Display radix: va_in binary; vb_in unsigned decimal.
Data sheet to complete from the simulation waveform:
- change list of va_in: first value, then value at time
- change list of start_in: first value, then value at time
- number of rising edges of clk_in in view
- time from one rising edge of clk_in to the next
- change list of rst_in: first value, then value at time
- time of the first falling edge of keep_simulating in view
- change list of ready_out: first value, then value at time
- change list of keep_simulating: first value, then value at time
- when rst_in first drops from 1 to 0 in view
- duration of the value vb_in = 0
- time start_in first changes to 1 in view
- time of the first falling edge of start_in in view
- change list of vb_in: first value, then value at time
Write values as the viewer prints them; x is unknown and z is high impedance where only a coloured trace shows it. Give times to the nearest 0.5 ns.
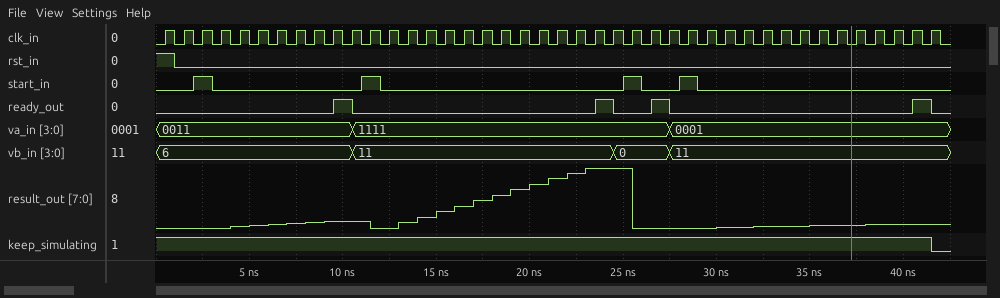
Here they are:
0011, 1111 at 10.5 ns, 0001 at 27.5 ns
0, 1 at 2 ns, 0 at 3 ns, 1 at 11 ns, 0 at 12 ns, 1 at 25 ns, 0 at 26 ns, 1 at 28 ns, 0 at 29 ns
42
1 ns
1, 0 at 1 ns
41.5 ns
0, 1 at 9.5 ns, 0 at 10.5 ns, 1 at 23.5 ns, 0 at 24.5 ns, 1 at 26.5 ns, 0 at 27.5 ns, 1 at 40.5 ns, 0 at 41.5 ns
1, 0 at 41.5 ns
1 ns
3 ns
2 ns
3 ns
6, 11 at 10.5 ns, 0 at 24.5 ns, 11 at 27.5 ns
